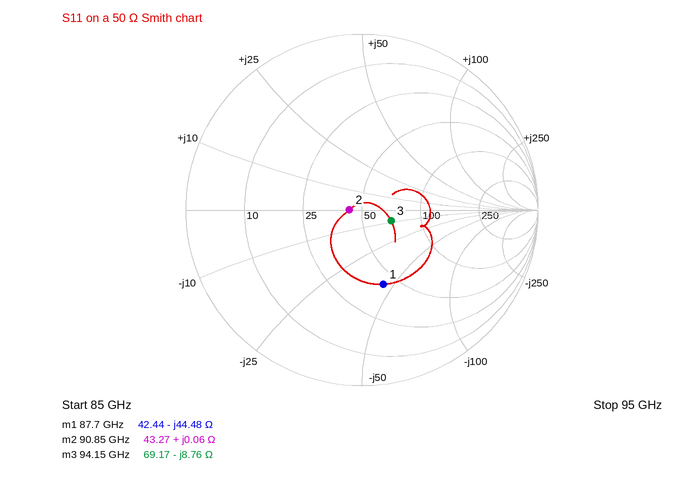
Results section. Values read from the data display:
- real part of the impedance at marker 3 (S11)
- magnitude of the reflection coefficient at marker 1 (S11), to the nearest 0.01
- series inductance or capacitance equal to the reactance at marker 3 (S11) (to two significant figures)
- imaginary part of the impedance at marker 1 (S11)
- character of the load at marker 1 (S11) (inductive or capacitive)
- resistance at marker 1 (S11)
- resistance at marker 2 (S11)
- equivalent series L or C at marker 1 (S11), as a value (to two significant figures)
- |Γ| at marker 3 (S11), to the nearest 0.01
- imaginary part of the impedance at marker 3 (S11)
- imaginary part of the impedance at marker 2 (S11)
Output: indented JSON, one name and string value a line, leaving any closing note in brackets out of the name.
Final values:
{
  "real part of the impedance at marker 3": "69.17 Ω",
  "magnitude of the reflection coefficient at marker 1 (S11), to the nearest 0.01": "0.44",
  "series inductance or capacitance equal to the reactance at marker 3 (S11)": "190 fF",
  "imaginary part of the impedance at marker 1": "-44.48 Ω",
  "character of the load at marker 1 (S11)": "capacitive",
  "resistance at marker 1": "42.44 Ω",
  "resistance at marker 2": "43.27 Ω",
  "equivalent series L or C at marker 1 (S11), as a value": "41 fF",
  "|Γ| at marker 3 (S11), to the nearest 0.01": "0.18",
  "imaginary part of the impedance at marker 3": "-8.76 Ω",
  "imaginary part of the impedance at marker 2": "+0.06 Ω"
}
